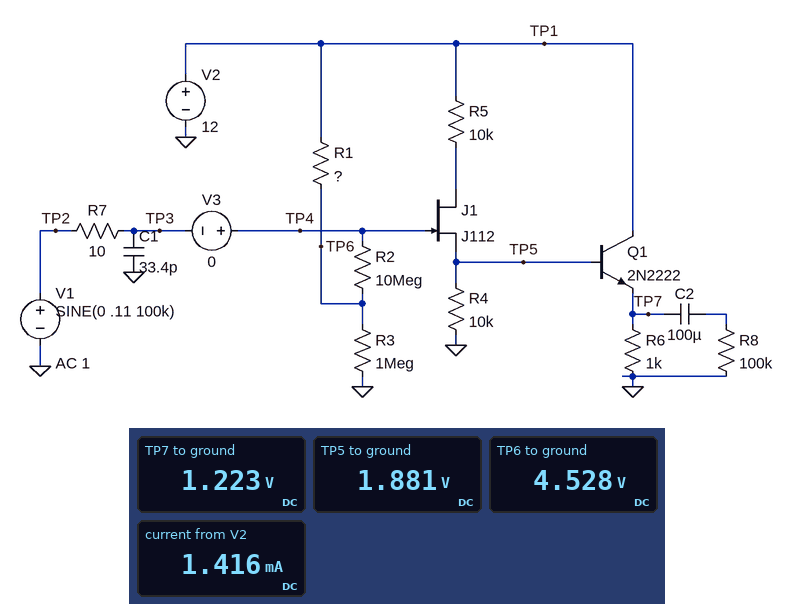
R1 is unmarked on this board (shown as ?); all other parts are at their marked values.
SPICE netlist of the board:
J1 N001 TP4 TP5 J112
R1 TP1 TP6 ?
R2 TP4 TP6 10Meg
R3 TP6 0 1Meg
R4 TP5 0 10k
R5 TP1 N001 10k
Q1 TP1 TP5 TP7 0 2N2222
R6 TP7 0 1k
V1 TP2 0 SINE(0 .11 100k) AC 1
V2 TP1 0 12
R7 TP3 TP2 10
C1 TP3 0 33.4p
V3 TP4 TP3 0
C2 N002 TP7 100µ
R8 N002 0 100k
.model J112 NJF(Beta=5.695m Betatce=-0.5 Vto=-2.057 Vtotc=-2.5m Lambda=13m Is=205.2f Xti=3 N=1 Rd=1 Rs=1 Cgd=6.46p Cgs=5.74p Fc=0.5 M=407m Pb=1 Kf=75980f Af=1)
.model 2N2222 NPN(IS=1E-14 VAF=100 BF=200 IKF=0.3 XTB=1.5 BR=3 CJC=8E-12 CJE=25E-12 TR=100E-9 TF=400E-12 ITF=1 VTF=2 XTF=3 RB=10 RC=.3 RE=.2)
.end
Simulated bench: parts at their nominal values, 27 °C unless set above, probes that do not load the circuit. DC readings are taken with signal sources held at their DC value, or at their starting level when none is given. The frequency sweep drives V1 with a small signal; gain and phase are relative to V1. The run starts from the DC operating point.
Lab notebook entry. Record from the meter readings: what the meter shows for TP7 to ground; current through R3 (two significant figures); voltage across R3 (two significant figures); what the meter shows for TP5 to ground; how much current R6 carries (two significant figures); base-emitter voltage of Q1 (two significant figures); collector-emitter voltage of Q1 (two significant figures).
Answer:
1.223 V
4.5 µA
4.5 V
1.881 V
1.2 mA
660 mV
11 V
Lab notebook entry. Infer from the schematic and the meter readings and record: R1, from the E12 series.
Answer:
1.5 MΩ
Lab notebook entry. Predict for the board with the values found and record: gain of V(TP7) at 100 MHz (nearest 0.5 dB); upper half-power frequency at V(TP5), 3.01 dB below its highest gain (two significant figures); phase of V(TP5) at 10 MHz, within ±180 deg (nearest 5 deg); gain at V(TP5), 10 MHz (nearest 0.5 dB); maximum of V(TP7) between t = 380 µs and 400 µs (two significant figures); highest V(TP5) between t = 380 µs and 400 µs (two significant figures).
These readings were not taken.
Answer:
-5.5 dB
56 MHz
-10 deg
-0.5 dB
1.3 V
2.0 V
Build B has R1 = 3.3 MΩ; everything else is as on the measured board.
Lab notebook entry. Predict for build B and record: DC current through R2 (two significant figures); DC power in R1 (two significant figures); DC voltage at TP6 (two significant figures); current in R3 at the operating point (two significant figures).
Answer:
260 nA
27 µW
2.6 V
2.6 µA
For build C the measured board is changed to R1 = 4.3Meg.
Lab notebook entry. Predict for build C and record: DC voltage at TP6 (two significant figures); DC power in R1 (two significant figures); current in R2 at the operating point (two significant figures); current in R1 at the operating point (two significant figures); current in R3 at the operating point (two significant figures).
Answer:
2.1 V
23 µW
210 nA
2.3 µA
2.1 µA
